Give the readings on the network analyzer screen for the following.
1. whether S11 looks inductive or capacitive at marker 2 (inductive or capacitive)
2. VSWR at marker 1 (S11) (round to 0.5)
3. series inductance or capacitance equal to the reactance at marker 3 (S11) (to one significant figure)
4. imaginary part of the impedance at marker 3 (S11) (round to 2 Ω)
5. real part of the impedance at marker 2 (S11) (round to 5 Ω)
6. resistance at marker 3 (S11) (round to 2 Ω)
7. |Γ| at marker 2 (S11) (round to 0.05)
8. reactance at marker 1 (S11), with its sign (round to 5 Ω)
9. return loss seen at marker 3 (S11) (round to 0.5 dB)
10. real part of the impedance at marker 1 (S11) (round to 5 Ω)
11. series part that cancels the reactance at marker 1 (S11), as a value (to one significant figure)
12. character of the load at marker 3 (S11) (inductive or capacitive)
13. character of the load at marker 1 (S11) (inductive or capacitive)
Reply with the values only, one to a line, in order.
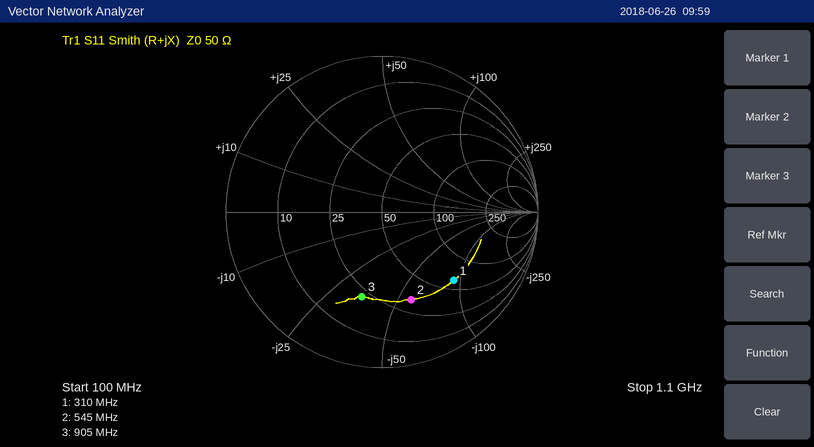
capacitive
4.5
5 pF
-34 Ω
35 Ω
22 Ω
0.60
-90 Ω
5.0 dB
60 Ω
50 nH
capacitive
capacitive
